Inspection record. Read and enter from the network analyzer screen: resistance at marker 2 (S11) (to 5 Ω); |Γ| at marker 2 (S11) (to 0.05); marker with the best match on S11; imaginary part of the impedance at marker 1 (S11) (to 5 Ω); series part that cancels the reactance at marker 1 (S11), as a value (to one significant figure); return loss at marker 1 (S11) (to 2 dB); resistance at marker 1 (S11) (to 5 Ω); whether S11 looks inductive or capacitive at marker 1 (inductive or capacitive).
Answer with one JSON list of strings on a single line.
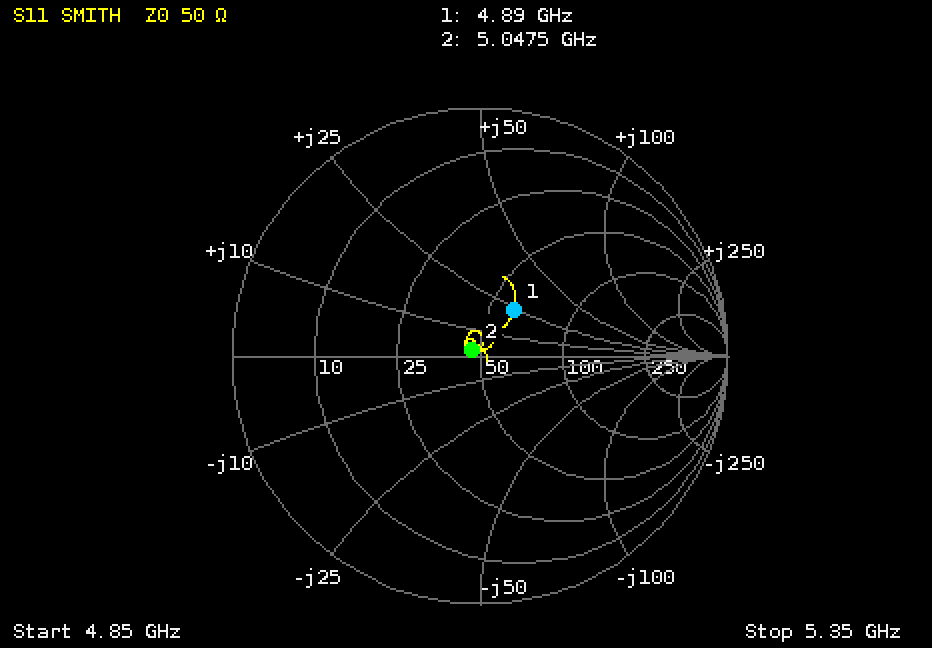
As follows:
["45 Ω", "0.05", "marker 2", "+25 Ω", "1 pF", "12 dB", "60 Ω", "inductive"]
